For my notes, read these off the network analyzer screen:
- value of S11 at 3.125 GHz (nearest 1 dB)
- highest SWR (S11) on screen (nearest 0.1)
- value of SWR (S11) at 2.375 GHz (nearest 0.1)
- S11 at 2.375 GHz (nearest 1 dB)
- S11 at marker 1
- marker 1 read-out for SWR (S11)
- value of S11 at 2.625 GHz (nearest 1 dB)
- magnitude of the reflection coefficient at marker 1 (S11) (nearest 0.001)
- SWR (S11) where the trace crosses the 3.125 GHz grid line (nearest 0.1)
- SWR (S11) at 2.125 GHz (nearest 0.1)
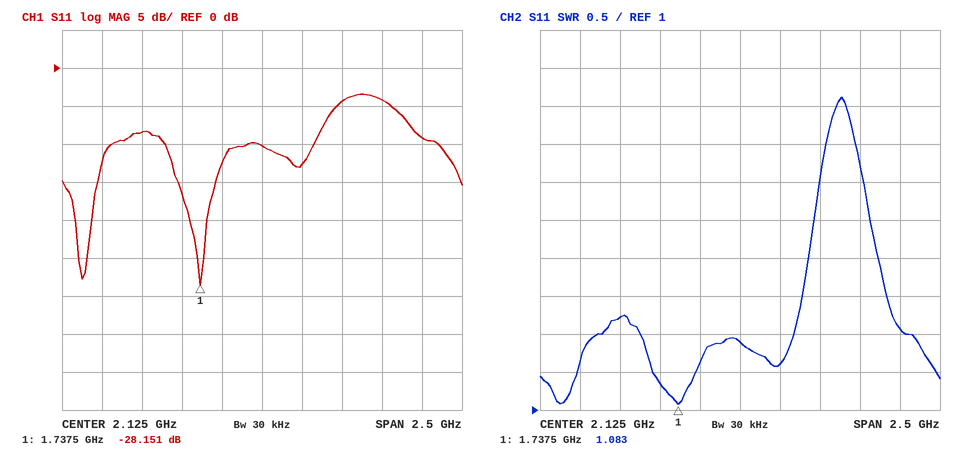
-9 dB
5.1
1.6
-13 dB
-28.151 dB
1.083
-4 dB
0.039
2.1
1.9
